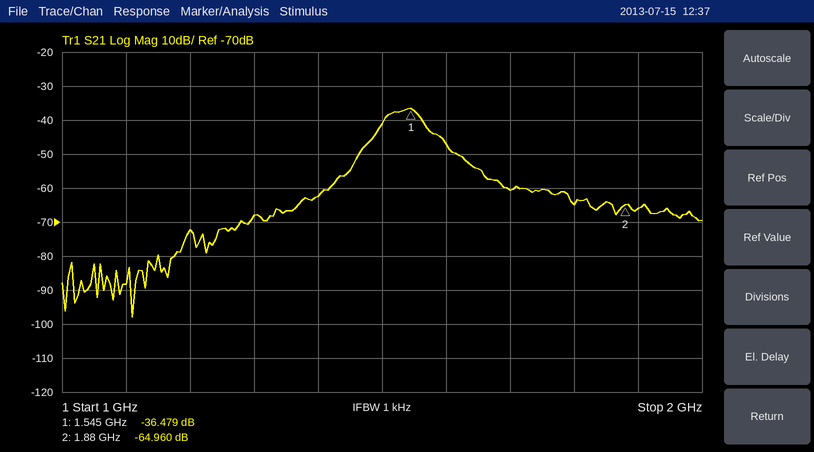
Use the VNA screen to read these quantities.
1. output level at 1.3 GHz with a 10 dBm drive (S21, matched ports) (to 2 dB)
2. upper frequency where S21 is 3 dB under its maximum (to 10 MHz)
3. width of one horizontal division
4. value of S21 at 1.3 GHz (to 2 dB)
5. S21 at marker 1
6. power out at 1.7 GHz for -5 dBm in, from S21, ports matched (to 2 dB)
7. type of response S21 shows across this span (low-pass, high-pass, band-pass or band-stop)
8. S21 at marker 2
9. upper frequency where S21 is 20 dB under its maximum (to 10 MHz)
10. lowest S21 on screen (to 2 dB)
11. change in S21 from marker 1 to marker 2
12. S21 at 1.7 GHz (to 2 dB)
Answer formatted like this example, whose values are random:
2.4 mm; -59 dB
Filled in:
-58 dBm; 1.56 GHz; 100 MHz; -68 dB; -36.479 dB; -66 dBm; band-pass; -64.960 dB; 1.66 GHz; -98 dB; -28.481 dB; -60 dB
